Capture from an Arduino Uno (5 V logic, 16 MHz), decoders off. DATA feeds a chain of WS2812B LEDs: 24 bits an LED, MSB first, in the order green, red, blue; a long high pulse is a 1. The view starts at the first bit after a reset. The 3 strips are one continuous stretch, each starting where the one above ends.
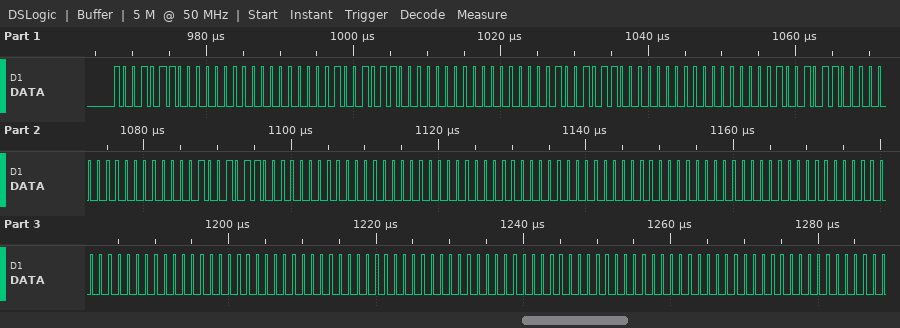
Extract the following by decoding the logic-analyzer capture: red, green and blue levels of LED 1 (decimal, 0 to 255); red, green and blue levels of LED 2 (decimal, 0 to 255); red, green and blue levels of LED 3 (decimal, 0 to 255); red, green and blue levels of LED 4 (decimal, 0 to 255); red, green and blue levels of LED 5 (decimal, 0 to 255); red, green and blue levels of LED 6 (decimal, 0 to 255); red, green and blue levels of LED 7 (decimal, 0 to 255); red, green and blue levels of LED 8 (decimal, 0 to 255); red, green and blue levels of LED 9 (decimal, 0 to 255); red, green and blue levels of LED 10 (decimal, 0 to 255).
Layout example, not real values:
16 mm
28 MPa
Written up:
0, 150, 0
0, 150, 0
0, 150, 0
0, 150, 0
0, 150, 0
0, 0, 0
0, 0, 0
0, 0, 0
0, 0, 0
0, 0, 0
